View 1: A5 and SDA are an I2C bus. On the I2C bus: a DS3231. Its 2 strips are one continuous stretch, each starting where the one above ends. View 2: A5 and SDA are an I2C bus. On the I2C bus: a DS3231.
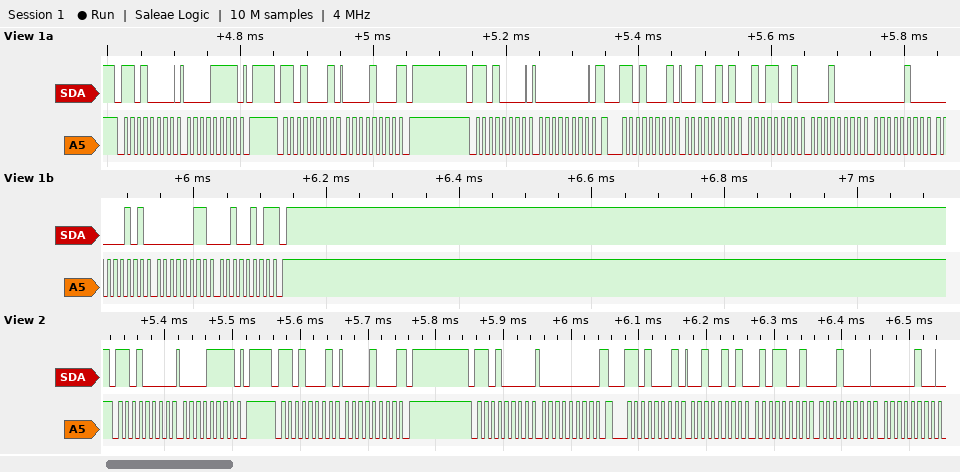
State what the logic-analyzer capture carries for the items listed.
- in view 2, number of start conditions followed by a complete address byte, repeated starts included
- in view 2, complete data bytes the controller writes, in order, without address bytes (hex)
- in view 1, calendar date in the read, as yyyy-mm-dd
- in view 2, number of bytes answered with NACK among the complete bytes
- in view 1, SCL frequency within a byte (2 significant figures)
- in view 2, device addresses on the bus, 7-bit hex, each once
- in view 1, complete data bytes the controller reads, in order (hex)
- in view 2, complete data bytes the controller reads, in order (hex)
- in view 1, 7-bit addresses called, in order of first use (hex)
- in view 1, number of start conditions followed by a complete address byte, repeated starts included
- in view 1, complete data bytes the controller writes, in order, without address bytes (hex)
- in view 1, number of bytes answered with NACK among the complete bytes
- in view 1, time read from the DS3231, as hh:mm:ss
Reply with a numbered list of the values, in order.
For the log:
1. 4
2. 0F 00
3. 2025-03-05
4. 1
5. 100 kHz
6. 0x68
7. 08 25 59 10 04 05 03 25
8. 08 25 59 10 04
9. 0x68
10. 4
11. 0F 00
12. 2
13. 10:59:25
